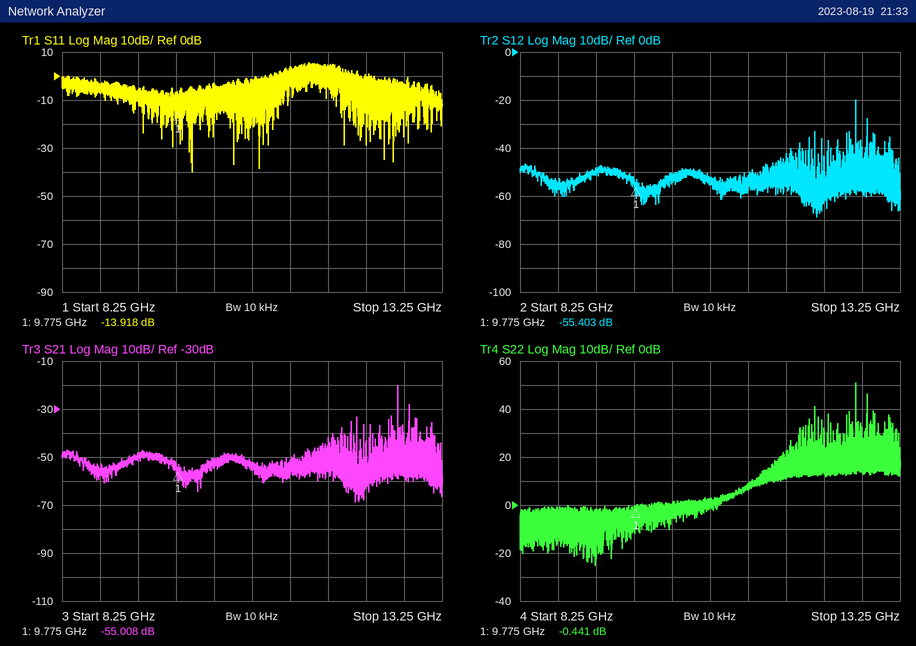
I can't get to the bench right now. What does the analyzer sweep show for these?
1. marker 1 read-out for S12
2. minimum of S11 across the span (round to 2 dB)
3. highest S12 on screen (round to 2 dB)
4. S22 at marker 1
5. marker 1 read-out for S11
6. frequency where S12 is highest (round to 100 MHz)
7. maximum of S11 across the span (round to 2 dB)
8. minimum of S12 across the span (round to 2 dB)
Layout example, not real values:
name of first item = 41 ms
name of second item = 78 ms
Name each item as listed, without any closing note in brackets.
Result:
marker 1 read-out for S12 = -55.403 dB
minimum of S11 across the span = -40 dB
highest S12 on screen = -20 dB
S22 at marker 1 = -0.441 dB
marker 1 read-out for S11 = -13.918 dB
frequency where S12 is highest = 12.7 GHz
maximum of S11 across the span = 6 dB
minimum of S12 across the span = -68 dB
